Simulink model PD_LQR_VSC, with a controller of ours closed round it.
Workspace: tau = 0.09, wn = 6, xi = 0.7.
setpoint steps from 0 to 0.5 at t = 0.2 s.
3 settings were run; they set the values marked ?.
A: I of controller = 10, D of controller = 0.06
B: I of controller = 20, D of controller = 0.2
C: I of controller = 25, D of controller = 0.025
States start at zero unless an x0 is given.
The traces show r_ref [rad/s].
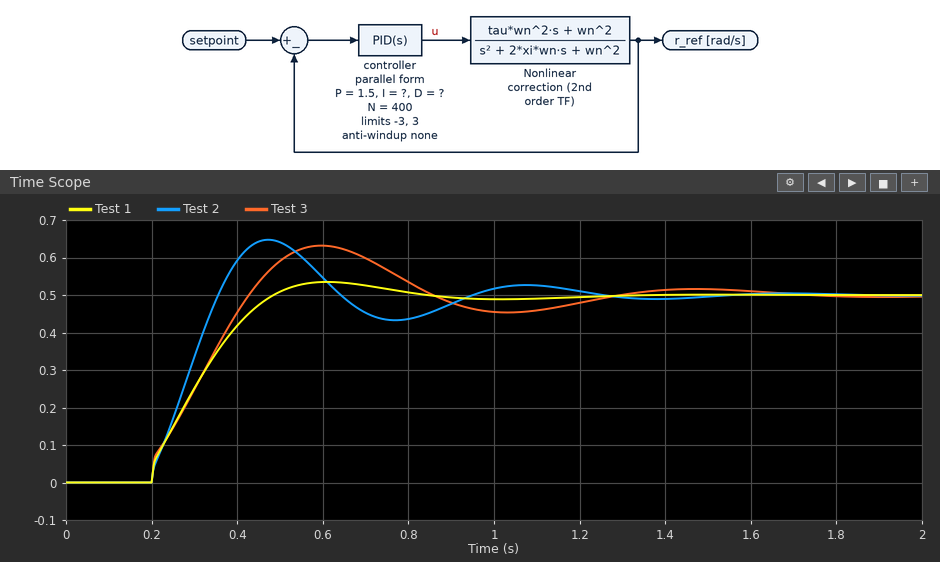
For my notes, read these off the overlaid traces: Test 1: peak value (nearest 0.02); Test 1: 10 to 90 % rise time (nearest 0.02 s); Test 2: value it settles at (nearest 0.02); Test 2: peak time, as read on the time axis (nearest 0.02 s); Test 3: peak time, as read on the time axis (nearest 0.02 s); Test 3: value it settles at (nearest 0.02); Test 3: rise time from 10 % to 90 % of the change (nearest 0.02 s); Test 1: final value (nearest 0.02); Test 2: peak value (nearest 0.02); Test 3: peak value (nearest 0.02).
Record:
0.54
0.22 s
0.50
0.48 s
0.60 s
0.50
0.20 s
0.50
0.64
0.64
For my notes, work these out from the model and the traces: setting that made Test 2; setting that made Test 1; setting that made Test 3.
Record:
C
A
B
